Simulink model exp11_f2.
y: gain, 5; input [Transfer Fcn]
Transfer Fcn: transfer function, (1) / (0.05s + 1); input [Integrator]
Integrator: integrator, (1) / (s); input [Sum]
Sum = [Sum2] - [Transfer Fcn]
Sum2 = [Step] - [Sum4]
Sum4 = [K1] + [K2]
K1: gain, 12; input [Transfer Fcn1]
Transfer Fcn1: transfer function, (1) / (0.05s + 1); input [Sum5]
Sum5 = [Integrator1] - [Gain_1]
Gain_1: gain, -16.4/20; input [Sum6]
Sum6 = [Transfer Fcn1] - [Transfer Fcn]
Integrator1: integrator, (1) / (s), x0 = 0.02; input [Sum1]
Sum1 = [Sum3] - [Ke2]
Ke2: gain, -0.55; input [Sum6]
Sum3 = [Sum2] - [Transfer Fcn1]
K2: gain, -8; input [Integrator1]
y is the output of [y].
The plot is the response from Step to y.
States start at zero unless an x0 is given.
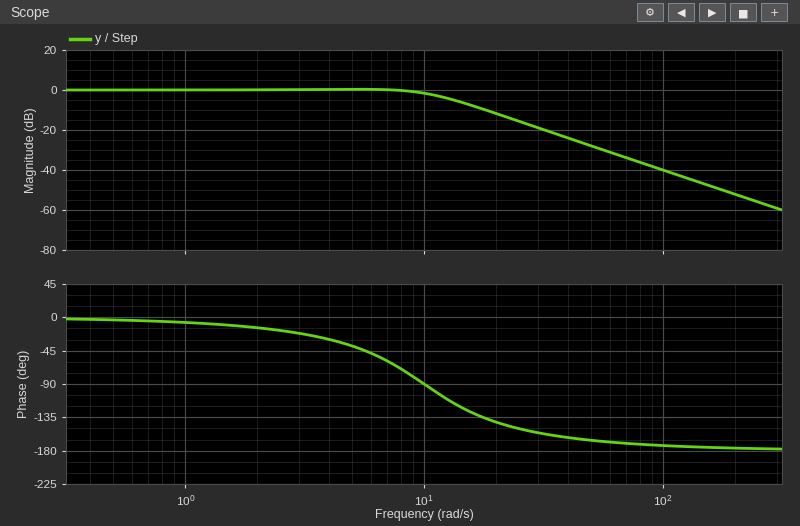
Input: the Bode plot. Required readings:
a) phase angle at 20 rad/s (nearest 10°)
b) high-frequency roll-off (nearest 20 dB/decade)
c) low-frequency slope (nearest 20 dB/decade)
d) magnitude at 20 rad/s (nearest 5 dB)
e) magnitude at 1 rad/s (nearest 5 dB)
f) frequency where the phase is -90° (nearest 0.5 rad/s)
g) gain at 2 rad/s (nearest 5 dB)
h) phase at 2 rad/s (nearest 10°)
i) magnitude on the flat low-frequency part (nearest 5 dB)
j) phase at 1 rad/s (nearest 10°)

-140°
-40 dB/decade
0 dB/decade
-10 dB
0 dB
10.0 rad/s
0 dB
-10°
0 dB
-10°
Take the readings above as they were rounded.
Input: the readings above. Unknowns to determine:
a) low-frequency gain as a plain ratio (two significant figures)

1.0
